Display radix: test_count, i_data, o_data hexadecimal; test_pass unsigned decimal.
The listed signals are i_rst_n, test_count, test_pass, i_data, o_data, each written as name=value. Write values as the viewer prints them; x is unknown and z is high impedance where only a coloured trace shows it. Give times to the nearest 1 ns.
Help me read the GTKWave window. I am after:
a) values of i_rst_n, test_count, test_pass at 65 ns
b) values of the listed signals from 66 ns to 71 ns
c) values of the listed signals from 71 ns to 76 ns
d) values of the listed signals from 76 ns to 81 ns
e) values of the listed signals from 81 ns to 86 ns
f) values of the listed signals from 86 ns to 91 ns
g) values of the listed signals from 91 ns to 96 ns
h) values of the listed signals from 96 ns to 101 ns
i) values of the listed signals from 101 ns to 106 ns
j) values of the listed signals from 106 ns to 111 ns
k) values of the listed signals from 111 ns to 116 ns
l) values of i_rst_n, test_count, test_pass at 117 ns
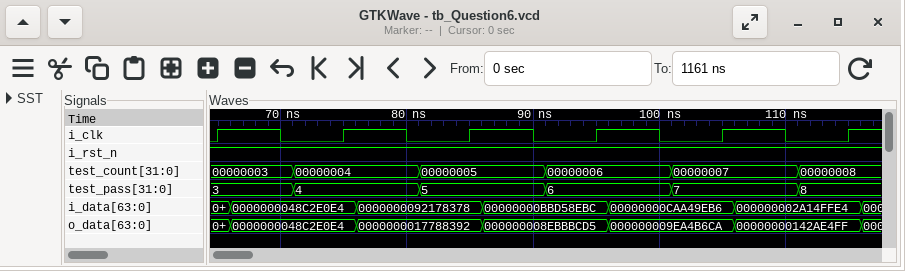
i_rst_n=1, test_count=00000003, test_pass=3
i_rst_n=1, test_count=00000003, test_pass=3, i_data=0000000048C2E0E4, o_data=0000000048C2E0E4
i_rst_n=1, test_count=00000004, test_pass=4, i_data=0000000048C2E0E4, o_data=0000000048C2E0E4
i_rst_n=1, test_count=00000004, test_pass=4, i_data=0000000092178378, o_data=0000000017788392
i_rst_n=1, test_count=00000005, test_pass=5, i_data=0000000092178378, o_data=0000000017788392
i_rst_n=1, test_count=00000005, test_pass=5, i_data=00000000BBD58EBC, o_data=000000008EBBBCD5
i_rst_n=1, test_count=00000006, test_pass=6, i_data=00000000BBD58EBC, o_data=000000008EBBBCD5
i_rst_n=1, test_count=00000006, test_pass=6, i_data=00000000CAA49EB6, o_data=000000009EA4B6CA
i_rst_n=1, test_count=00000007, test_pass=7, i_data=00000000CAA49EB6, o_data=000000009EA4B6CA
i_rst_n=1, test_count=00000007, test_pass=7, i_data=000000002A14FFE4, o_data=00000000142AE4FF
i_rst_n=1, test_count=00000008, test_pass=8, i_data=000000002A14FFE4, o_data=00000000142AE4FF
i_rst_n=1, test_count=00000008, test_pass=8
